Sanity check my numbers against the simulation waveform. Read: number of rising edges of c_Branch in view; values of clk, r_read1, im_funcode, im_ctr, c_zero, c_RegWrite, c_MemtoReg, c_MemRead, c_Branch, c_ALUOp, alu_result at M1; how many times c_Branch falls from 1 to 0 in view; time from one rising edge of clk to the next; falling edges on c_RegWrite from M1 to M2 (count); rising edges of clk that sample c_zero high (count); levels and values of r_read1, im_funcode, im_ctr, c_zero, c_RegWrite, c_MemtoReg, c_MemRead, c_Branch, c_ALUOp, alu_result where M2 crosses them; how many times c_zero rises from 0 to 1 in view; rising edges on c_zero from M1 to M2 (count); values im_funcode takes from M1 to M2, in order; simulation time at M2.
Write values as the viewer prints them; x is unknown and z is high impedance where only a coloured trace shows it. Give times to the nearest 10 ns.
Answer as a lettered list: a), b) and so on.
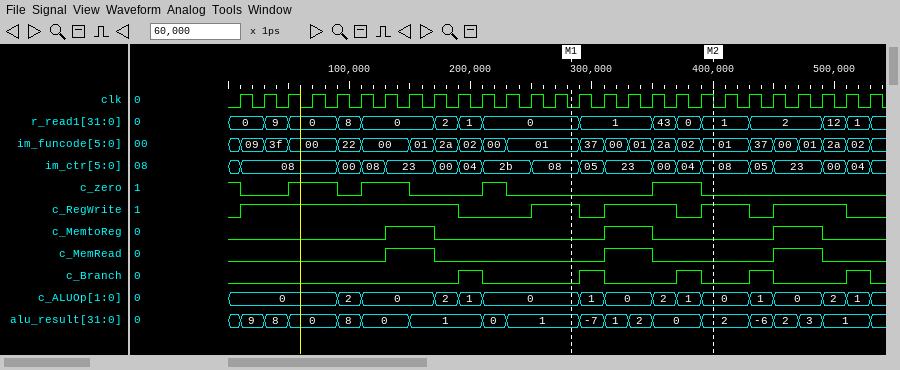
a) 5
b) clk=0, r_read1=0, im_funcode=01, im_ctr=08, c_zero=0, c_RegWrite=1, c_MemtoReg=0, c_MemRead=0, c_Branch=0, c_ALUOp=0, alu_result=1
c) 5
d) 20 ns
e) 2
f) 8
g) r_read1=1, im_funcode=01, im_ctr=08, c_zero=0, c_RegWrite=1, c_MemtoReg=0, c_MemRead=0, c_Branch=0, c_ALUOp=0, alu_result=2
h) 4
i) 1
j) 01, 37, 00, 01, 2a, 02, 01
k) 400 ns
